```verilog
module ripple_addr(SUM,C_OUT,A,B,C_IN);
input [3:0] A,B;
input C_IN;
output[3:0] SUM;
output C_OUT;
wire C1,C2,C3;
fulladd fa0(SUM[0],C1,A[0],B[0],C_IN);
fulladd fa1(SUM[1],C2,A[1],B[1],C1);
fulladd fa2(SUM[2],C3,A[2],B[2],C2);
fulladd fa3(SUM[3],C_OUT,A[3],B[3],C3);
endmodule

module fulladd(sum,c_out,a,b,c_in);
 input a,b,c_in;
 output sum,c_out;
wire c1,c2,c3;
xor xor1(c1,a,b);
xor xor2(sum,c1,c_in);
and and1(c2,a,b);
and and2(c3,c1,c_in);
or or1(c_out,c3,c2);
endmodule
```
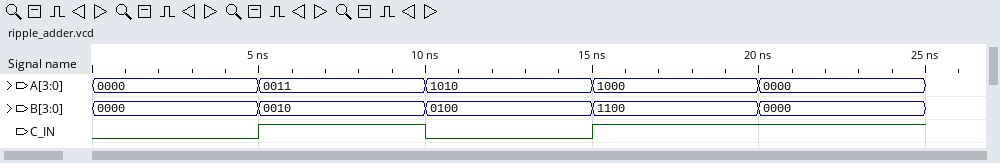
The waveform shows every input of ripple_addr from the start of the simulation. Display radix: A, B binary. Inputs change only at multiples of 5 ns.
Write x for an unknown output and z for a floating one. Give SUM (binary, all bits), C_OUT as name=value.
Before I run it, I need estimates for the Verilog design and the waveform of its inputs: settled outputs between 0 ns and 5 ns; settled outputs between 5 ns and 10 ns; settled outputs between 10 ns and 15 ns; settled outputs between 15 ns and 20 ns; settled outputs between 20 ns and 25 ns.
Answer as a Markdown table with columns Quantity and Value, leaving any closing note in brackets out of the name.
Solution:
| Quantity | Value |
|---|---|
| settled outputs between 0 ns and 5 ns | SUM=0000, C_OUT=0 |
| settled outputs between 5 ns and 10 ns | SUM=0110, C_OUT=0 |
| settled outputs between 10 ns and 15 ns | SUM=1110, C_OUT=0 |
| settled outputs between 15 ns and 20 ns | SUM=0101, C_OUT=1 |
| settled outputs between 20 ns and 25 ns | SUM=0001, C_OUT=0 |
